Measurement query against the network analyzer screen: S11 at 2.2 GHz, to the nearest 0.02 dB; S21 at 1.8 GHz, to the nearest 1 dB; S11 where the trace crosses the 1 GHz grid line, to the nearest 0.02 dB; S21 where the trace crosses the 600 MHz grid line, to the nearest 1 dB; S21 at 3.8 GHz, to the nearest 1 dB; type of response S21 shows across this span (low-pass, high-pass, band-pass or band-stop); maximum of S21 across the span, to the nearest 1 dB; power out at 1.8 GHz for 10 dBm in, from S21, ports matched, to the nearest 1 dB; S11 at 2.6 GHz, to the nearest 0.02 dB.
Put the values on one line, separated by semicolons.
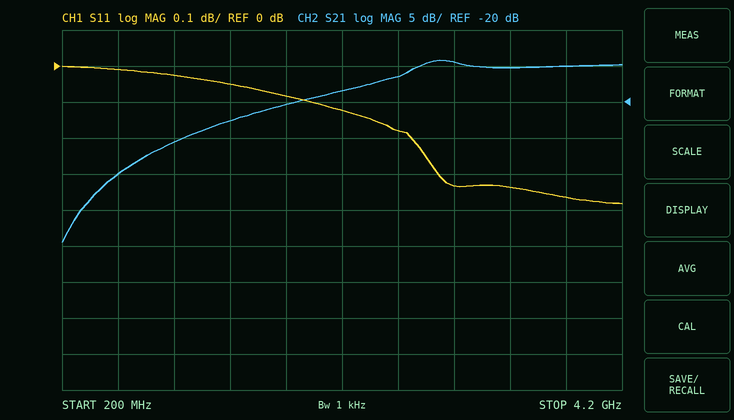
-0.12 dB; -20 dB; -0.02 dB; -30 dB; -15 dB; high-pass; -14 dB; -10 dBm; -0.18 dB
